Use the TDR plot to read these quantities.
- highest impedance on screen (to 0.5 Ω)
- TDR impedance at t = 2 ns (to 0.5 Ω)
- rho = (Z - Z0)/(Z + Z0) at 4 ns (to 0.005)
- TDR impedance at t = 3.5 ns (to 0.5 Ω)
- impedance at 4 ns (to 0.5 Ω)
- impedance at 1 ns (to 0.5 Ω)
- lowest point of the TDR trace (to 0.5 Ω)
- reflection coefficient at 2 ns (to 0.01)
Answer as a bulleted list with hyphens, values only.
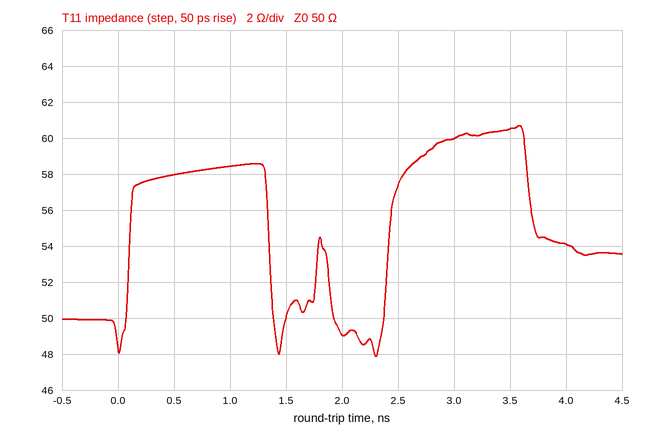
- 60.5 Ω
- 49.0 Ω
- +0.040
- 60.5 Ω
- 54.0 Ω
- 58.5 Ω
- 48.0 Ω
- -0.01
